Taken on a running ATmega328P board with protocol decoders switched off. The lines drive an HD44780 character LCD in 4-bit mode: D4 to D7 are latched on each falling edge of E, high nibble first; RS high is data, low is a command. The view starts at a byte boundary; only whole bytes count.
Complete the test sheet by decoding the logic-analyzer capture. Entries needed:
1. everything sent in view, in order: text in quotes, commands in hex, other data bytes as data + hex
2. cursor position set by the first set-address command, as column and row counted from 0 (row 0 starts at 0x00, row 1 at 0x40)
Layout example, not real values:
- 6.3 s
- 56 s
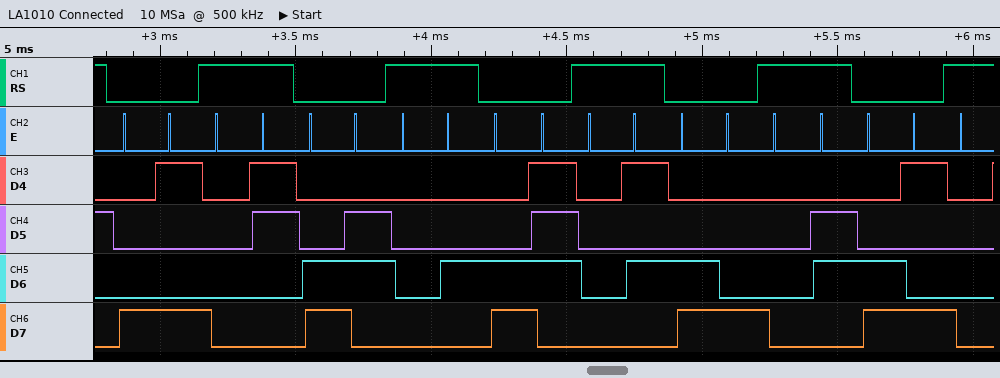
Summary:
- 0x89 data 03 0xC6 data 04 0xC7 data 05 0xC8 data 06 0xC9
- column 9, row 0
